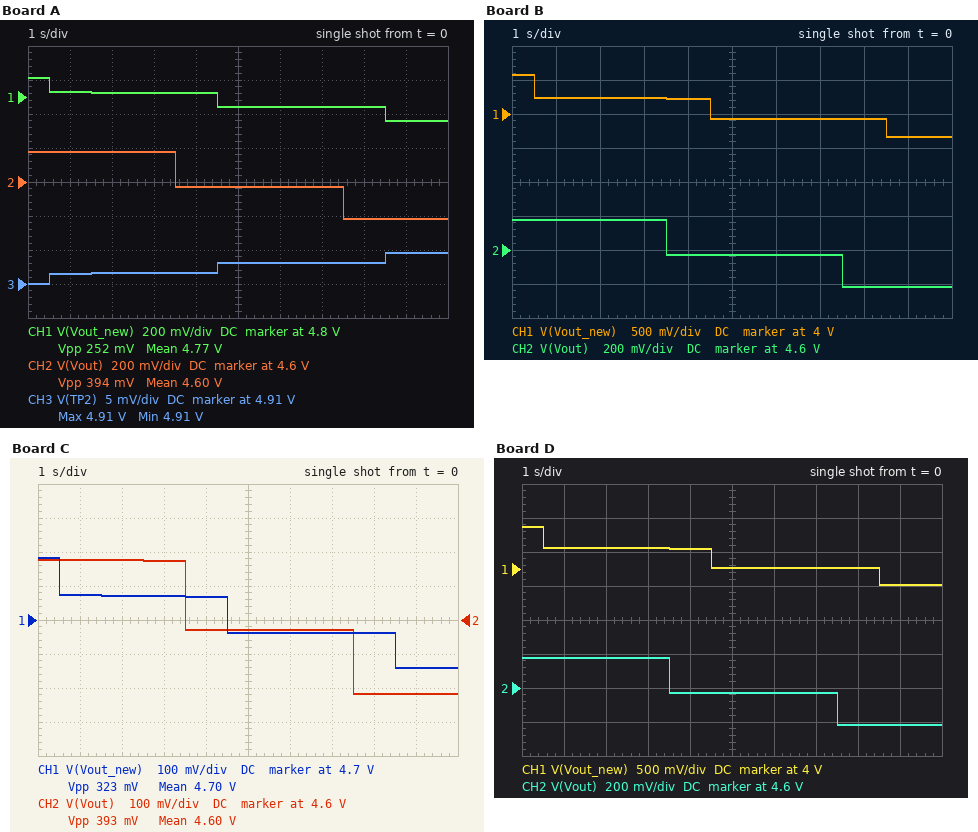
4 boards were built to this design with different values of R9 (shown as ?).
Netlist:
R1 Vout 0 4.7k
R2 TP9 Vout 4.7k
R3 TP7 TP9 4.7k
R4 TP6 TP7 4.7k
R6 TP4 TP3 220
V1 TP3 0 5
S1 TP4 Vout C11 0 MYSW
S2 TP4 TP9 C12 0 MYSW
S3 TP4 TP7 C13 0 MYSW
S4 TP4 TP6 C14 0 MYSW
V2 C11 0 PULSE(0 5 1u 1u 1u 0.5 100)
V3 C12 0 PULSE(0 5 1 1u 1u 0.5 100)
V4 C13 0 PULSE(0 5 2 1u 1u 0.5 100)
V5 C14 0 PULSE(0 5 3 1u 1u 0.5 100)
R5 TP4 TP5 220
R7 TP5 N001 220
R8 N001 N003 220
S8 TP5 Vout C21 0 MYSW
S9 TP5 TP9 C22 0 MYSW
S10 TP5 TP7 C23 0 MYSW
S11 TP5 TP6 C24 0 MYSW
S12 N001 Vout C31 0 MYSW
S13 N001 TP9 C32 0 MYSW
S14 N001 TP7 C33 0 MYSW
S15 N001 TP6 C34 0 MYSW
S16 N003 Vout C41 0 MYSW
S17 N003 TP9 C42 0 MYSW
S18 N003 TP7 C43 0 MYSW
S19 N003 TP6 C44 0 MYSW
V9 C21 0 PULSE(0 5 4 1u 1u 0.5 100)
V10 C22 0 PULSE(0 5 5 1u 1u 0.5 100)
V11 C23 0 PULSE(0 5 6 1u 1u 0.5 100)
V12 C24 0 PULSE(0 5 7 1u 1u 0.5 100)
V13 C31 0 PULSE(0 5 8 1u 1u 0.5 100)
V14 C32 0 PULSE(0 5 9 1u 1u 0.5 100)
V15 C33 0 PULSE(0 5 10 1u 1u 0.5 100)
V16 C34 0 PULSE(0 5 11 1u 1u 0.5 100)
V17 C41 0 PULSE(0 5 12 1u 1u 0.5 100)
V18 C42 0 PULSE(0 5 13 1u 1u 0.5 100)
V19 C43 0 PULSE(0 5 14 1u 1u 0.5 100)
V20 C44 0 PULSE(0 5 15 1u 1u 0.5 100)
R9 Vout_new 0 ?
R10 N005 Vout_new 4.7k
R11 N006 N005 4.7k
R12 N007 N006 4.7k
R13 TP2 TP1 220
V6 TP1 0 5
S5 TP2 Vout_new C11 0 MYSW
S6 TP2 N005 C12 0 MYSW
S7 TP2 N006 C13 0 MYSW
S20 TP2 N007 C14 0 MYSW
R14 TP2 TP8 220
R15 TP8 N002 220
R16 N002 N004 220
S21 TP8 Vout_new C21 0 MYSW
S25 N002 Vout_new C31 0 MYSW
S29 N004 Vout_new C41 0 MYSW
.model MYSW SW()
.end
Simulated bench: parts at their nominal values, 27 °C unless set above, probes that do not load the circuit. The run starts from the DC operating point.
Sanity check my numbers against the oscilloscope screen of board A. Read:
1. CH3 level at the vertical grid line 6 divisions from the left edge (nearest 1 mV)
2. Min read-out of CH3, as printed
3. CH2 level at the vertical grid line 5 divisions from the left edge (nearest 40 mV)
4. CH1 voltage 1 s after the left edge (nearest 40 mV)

4.913 V
4.91 V
4.56 V
4.84 V
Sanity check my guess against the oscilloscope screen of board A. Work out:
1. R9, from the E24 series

12 kΩ
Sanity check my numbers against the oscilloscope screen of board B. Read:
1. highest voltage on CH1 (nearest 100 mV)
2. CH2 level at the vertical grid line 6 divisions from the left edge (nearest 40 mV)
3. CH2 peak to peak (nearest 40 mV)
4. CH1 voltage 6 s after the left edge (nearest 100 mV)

4.6 V
4.56 V
400 mV
3.9 V
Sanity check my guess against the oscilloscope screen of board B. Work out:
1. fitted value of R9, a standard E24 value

2.4 kΩ
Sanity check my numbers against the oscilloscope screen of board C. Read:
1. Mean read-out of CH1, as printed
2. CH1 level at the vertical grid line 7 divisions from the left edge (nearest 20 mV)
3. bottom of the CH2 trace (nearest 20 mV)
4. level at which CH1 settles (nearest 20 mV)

4.70 V
4.66 V
4.38 V
4.56 V
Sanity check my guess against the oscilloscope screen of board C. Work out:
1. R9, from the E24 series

9.1 kΩ
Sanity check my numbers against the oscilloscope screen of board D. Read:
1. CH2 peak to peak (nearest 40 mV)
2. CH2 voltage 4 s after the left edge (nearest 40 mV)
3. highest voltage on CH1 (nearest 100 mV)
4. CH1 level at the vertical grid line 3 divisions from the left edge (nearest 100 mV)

400 mV
4.56 V
4.6 V
4.3 V
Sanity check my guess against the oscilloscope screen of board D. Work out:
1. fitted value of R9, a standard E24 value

2.7 kΩ
